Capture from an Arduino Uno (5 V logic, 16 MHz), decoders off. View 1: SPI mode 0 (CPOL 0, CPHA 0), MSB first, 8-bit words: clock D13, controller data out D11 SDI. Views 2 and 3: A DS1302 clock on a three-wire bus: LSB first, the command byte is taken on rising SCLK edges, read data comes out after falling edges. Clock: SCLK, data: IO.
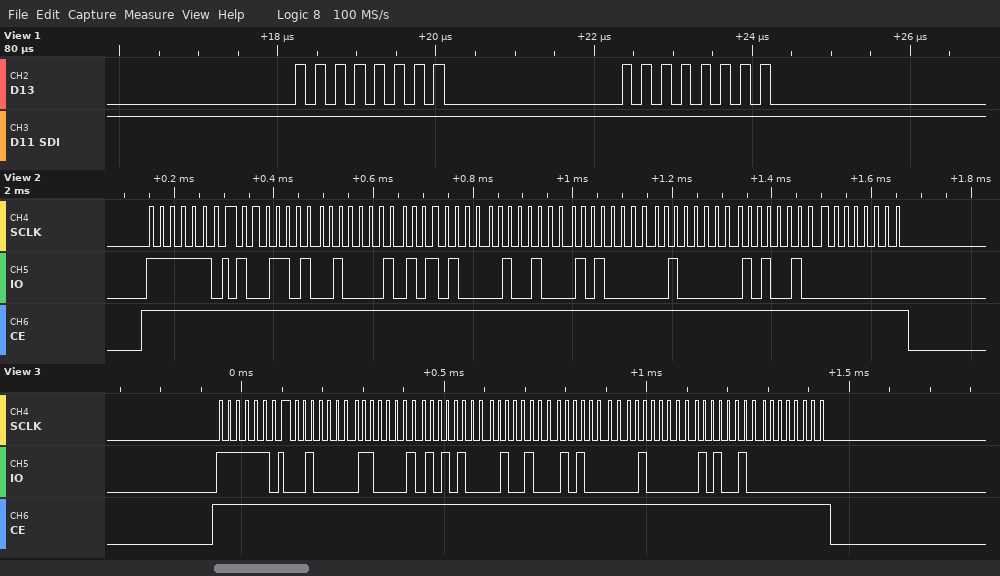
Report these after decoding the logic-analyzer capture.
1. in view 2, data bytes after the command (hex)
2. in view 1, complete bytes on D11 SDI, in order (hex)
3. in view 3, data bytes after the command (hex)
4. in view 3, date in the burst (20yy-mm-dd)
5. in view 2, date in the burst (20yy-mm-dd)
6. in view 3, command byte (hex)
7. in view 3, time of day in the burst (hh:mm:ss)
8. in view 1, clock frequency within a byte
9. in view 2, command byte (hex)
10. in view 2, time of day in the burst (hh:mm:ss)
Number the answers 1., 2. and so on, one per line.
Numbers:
1. 59 42 15 12 05 02 25 00
2. FF FF
3. 04 43 15 12 05 02 25 00
4. 2025-05-12
5. 2025-05-12
6. 0xBF
7. 15:43:04
8. 4 MHz
9. 0xBF
10. 15:42:59
